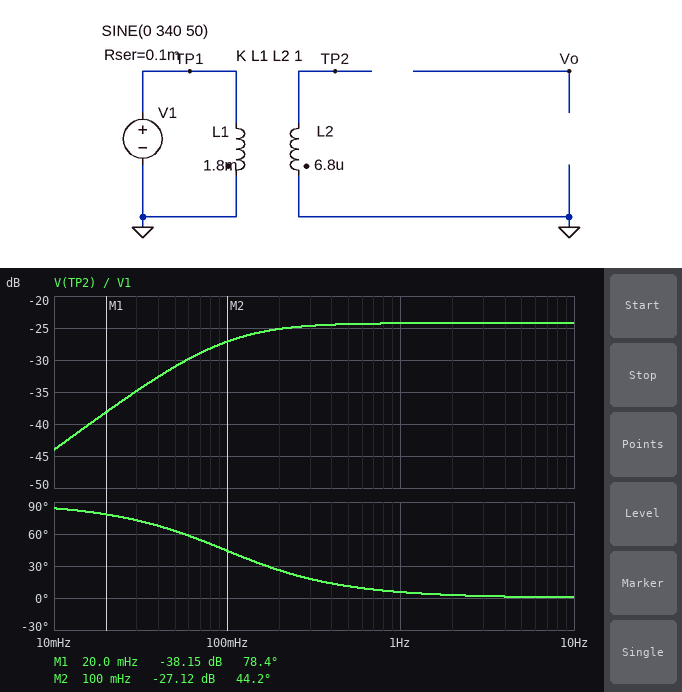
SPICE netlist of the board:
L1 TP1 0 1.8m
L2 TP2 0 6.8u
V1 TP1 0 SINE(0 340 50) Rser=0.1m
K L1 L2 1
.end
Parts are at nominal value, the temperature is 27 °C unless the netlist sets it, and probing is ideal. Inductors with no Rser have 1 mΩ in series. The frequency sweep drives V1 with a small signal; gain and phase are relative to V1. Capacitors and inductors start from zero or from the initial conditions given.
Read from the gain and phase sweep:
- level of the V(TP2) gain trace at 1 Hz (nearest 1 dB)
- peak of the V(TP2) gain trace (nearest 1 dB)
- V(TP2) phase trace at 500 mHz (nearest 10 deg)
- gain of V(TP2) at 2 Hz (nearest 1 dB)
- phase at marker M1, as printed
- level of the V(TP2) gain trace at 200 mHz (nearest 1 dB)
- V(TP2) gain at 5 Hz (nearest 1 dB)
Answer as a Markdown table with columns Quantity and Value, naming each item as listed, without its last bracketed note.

| Quantity | Value |
|---|---|
| level of the V(TP2) gain trace at 1 Hz | -24 dB |
| peak of the V(TP2) gain trace | -24 dB |
| V(TP2) phase trace at 500 mHz | 10 deg |
| gain of V(TP2) at 2 Hz | -24 dB |
| phase at marker M1, as printed | 78.4 deg |
| level of the V(TP2) gain trace at 200 mHz | -25 dB |
| V(TP2) gain at 5 Hz | -24 dB |
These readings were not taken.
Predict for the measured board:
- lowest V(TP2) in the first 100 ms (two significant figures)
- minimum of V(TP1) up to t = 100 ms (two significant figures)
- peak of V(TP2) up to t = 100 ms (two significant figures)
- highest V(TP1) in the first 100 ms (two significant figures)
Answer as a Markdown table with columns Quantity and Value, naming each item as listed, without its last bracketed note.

| Quantity | Value |
|---|---|
| lowest V(TP2) in the first 100 ms | -21 V |
| minimum of V(TP1) up to t = 100 ms | -340 V |
| peak of V(TP2) up to t = 100 ms | 21 V |
| highest V(TP1) in the first 100 ms | 340 V |
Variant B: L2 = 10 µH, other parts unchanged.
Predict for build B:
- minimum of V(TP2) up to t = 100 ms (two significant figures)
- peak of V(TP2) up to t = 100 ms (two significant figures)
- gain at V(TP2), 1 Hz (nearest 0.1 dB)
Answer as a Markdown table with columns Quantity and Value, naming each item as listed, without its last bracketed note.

| Quantity | Value |
|---|---|
| minimum of V(TP2) up to t = 100 ms | -25 V |
| peak of V(TP2) up to t = 100 ms | 25 V |
| gain at V(TP2), 1 Hz | -22.6 dB |
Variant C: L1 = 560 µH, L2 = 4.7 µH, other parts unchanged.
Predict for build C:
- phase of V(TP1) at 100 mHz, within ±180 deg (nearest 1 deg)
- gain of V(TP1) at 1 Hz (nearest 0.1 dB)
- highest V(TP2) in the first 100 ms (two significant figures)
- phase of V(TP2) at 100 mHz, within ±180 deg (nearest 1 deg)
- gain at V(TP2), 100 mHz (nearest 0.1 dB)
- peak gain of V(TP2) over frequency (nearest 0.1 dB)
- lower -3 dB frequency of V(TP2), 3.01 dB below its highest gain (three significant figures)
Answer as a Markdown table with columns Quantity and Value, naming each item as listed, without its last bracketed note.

| Quantity | Value |
|---|---|
| phase of V(TP1) at 100 mHz, within ±180 deg | 2 deg |
| gain of V(TP1) at 1 Hz | -0.1 dB |
| highest V(TP2) in the first 100 ms | 31 V |
| phase of V(TP2) at 100 mHz, within ±180 deg | 72 deg |
| gain at V(TP2), 100 mHz | -31.1 dB |
| peak gain of V(TP2) over frequency | -20.8 dB |
| lower -3 dB frequency of V(TP2), 3.01 dB below its highest gain | 313 mHz |
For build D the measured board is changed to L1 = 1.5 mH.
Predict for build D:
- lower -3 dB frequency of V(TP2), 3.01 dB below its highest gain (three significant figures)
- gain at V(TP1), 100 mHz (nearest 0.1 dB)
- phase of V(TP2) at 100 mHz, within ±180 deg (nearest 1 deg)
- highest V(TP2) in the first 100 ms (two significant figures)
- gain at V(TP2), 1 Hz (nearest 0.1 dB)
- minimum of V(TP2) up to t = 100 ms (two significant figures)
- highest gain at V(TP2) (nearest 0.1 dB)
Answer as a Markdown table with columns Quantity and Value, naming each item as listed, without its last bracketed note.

| Quantity | Value |
|---|---|
| lower -3 dB frequency of V(TP2), 3.01 dB below its highest gain | 117 mHz |
| gain at V(TP1), 100 mHz | -0.5 dB |
| phase of V(TP2) at 100 mHz, within ±180 deg | 49 deg |
| highest V(TP2) in the first 100 ms | 23 V |
| gain at V(TP2), 1 Hz | -23.5 dB |
| minimum of V(TP2) up to t = 100 ms | -23 V |
| highest gain at V(TP2) | -23.4 dB |
